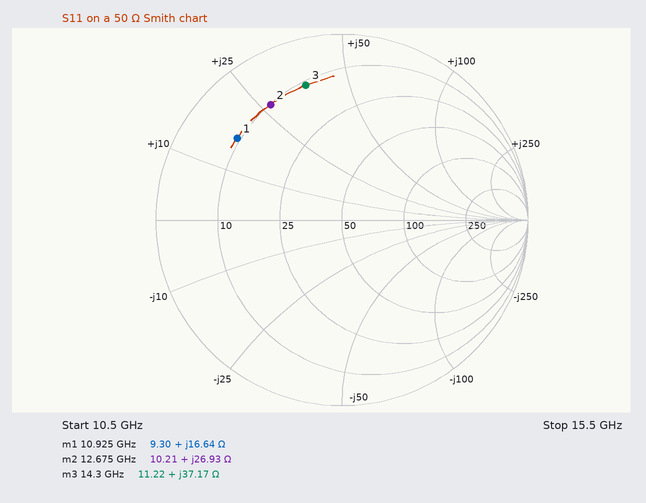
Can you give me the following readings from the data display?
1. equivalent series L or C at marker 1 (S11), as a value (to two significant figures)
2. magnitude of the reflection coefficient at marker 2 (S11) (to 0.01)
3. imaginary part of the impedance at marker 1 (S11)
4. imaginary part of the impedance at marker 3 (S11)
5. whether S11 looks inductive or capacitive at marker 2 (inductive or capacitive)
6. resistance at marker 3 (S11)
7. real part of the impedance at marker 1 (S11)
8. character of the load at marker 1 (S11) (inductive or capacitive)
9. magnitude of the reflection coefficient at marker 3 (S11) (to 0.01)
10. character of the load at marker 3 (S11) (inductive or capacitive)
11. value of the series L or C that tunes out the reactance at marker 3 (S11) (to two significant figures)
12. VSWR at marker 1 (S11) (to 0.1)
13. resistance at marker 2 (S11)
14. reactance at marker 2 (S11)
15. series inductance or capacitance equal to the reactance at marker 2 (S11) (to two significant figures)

240 pH
0.73
+16.64 Ω
+37.17 Ω
inductive
11.22 Ω
9.30 Ω
inductive
0.75
inductive
300 fF
6.0
10.21 Ω
+26.93 Ω
340 pH
